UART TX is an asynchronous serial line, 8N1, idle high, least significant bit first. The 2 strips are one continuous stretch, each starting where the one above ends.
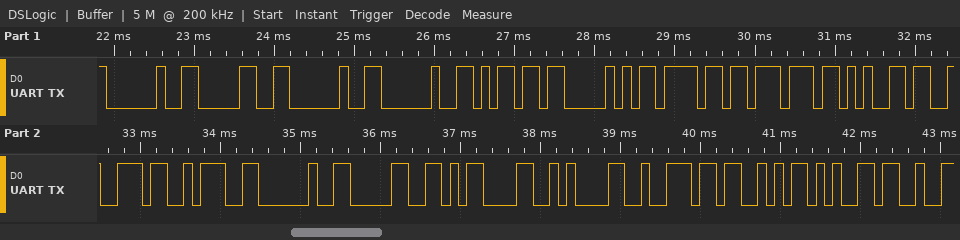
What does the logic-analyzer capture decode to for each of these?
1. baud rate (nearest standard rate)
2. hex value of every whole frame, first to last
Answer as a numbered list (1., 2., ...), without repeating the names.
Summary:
1. 9600 baud
2. 20 30 20 20 6D 50 6F 77 65 72 3A 20 30 0D 0A 72 53 65
